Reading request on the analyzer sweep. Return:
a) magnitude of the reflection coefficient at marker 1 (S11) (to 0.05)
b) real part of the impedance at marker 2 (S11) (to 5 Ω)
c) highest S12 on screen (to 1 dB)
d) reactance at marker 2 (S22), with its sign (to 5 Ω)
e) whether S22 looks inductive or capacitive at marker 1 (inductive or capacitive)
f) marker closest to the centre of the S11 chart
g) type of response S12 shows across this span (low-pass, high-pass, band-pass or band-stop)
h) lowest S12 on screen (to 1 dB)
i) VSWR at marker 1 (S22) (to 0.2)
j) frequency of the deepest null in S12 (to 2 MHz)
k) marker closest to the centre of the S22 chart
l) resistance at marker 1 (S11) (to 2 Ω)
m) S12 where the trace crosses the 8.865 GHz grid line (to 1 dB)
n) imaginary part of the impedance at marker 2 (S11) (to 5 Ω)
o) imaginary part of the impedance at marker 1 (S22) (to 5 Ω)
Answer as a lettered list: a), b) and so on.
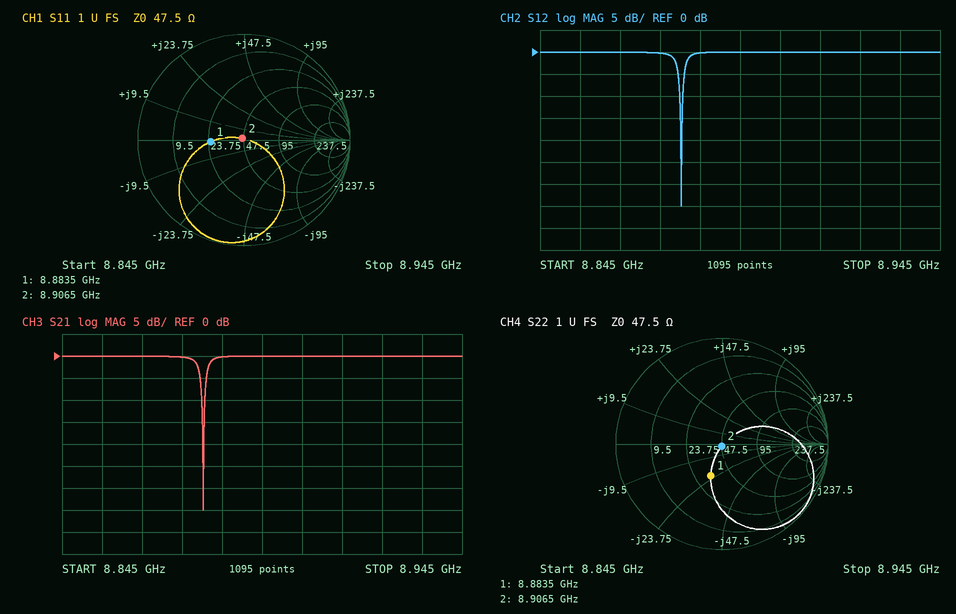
a) 0.30
b) 45 Ω
c) 0 dB
d) 0 Ω
e) capacitive
f) marker 2
g) band-stop
h) -35 dB
i) 2.0
j) 8.880 GHz
k) marker 2
l) 24 Ω
m) 0 dB
n) 0 Ω
o) -20 Ω
